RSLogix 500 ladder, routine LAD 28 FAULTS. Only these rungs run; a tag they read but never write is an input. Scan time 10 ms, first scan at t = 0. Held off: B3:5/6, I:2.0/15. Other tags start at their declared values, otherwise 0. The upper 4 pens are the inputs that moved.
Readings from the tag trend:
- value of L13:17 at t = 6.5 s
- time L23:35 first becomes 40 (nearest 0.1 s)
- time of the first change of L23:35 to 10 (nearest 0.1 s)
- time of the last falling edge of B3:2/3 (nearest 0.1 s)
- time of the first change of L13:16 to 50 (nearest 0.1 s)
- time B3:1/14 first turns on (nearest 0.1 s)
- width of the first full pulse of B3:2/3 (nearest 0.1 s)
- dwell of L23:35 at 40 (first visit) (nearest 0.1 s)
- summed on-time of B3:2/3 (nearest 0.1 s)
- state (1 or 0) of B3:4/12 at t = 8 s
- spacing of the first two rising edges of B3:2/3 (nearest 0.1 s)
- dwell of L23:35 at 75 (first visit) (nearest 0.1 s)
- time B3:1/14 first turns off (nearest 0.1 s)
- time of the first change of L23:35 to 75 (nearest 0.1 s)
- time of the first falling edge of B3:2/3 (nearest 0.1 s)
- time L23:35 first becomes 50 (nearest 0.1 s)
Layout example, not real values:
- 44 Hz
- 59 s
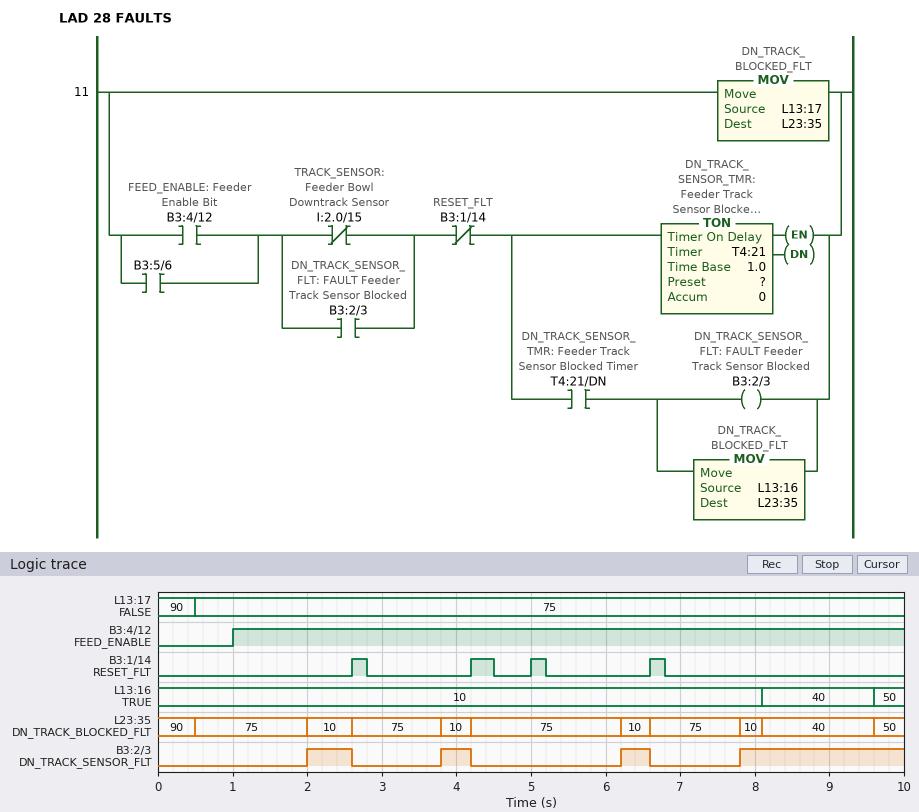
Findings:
- 75
- 8.1 s
- 2.0 s
- 6.6 s
- 9.6 s
- 2.6 s
- 0.6 s
- 1.5 s
- 3.6 s
- 1
- 1.8 s
- 1.5 s
- 2.8 s
- 0.5 s
- 2.6 s
- 9.6 s
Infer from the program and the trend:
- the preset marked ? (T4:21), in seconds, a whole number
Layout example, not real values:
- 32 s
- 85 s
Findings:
- 1 s
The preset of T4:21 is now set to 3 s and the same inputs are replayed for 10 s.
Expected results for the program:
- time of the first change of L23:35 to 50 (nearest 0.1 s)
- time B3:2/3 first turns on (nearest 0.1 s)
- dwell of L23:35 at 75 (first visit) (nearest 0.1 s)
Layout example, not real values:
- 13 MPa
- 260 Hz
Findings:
- 9.8 s
- 9.8 s
- 9.3 s
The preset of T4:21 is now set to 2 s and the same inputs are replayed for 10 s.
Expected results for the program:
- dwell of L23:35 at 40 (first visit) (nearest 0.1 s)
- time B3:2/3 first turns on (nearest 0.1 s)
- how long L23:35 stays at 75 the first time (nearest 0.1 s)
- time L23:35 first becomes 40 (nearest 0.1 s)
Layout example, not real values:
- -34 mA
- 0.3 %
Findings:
- 0.8 s
- 8.8 s
- 8.3 s
- 8.8 s
